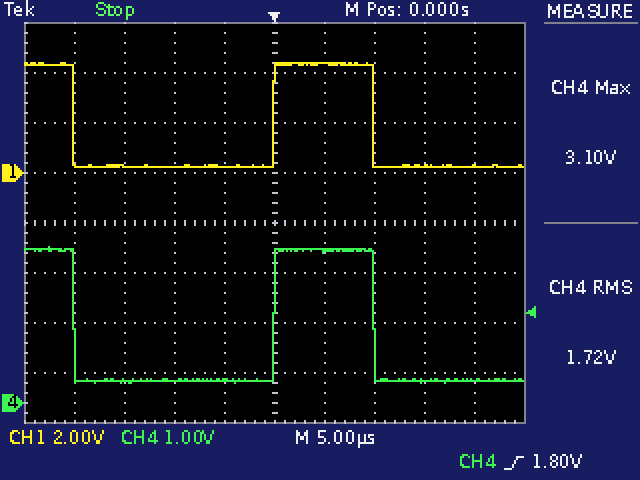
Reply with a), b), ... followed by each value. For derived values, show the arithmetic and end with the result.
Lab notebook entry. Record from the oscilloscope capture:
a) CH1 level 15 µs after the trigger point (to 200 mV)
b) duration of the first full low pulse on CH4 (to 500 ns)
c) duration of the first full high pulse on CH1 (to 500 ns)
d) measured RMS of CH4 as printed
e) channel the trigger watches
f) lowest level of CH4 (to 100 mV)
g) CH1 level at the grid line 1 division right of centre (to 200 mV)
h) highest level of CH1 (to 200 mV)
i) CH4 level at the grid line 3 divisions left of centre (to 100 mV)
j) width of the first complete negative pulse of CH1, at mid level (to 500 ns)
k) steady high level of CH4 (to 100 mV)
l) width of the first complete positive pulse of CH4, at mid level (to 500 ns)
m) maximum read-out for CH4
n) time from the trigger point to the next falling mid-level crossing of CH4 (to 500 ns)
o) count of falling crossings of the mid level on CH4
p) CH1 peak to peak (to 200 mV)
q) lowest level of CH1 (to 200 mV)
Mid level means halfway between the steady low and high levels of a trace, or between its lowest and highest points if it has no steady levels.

a) 200 mV
b) 20.0 µs
c) 10.0 µs
d) 1.72 V
e) CH4
f) 400 mV
g) 4.4 V
h) 4.4 V
i) 400 mV
j) 20.0 µs
k) 3.1 V
l) 10.0 µs
m) 3.10 V
n) 10.0 µs
o) 2
p) 4.4 V − (200 mV) = 4.2 V
q) 200 mV
